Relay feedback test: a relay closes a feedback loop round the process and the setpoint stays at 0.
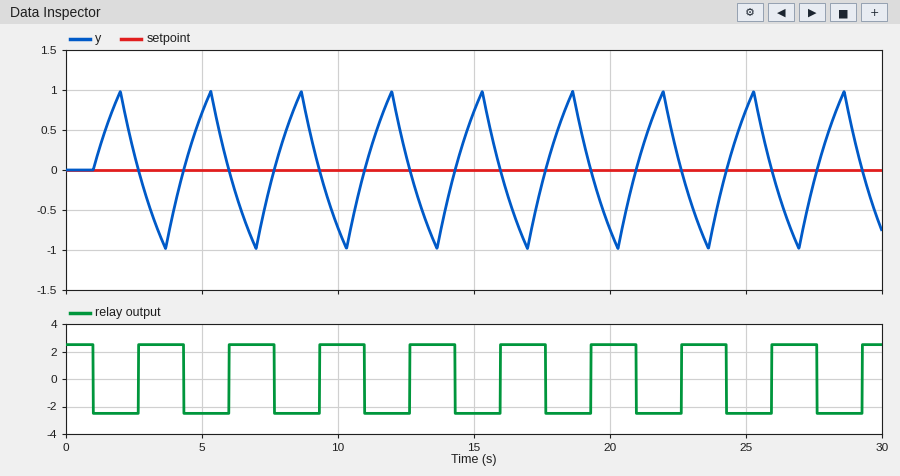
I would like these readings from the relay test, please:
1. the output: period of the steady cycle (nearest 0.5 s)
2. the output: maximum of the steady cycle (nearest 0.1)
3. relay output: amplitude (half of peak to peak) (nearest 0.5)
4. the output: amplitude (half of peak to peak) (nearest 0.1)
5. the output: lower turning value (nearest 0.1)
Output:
3.5 s
1.0
2.5
1.0
-1.0
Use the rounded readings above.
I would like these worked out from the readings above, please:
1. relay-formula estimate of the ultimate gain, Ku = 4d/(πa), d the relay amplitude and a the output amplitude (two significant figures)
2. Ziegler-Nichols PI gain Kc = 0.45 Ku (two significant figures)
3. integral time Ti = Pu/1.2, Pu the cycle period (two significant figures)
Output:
3.2
1.4
2.9 s
